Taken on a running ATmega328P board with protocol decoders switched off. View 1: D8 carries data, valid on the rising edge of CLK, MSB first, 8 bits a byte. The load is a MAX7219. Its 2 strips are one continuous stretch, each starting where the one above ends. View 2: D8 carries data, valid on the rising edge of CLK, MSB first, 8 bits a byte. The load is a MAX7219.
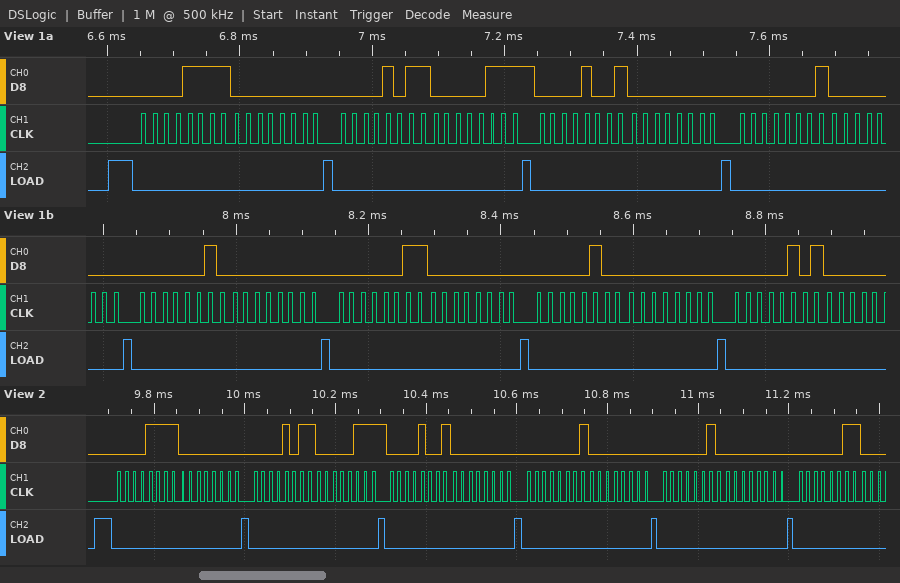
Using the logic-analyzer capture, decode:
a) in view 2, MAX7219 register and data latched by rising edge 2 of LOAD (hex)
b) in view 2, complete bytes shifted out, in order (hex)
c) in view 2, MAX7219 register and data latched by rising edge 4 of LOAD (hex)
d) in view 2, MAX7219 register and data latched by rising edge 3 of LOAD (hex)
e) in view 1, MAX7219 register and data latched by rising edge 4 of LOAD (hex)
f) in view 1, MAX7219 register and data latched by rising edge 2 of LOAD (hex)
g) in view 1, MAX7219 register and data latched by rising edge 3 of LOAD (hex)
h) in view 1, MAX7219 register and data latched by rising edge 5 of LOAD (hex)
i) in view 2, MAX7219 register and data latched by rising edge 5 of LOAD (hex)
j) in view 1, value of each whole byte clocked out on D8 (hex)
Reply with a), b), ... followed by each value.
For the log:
a) register 0xF, data 0x00
b) 0F 00 0B 07 09 00 01 00 02 00 03
c) register 0x9, data 0x00
d) register 0xB, data 0x07
e) register 0x9, data 0x00
f) register 0xF, data 0x00
g) register 0xB, data 0x07
h) register 0x1, data 0x00
i) register 0x1, data 0x00
j) 0x0F 0x00 0x0B 0x07 0x09 0x00 0x01 0x00 0x02 0x00 0x03 0x00 0x04 0x00 0x05
